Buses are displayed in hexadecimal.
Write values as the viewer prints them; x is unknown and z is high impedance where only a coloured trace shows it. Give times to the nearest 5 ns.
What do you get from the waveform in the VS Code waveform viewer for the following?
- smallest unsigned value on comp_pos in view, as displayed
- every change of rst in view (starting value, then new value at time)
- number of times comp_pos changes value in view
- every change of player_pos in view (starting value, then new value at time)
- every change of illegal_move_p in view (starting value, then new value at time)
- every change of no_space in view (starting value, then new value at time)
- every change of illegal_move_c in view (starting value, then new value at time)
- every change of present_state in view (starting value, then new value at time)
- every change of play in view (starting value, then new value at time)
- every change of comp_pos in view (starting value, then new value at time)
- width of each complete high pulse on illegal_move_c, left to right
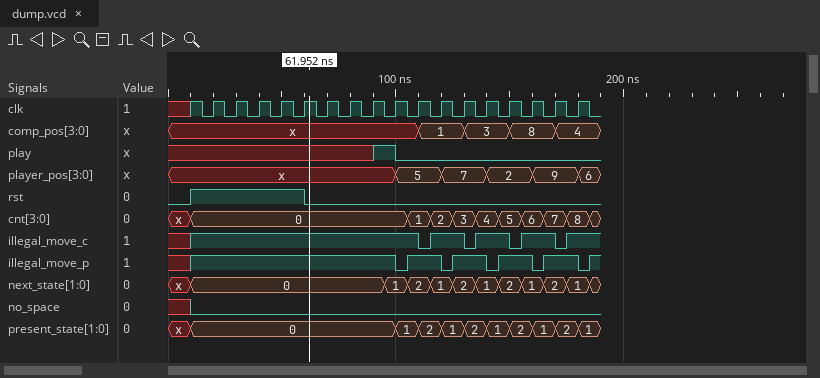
1
0, 1 at 10 ns, 0 at 60 ns
4
x, 5 at 100 ns, 7 at 120 ns, 2 at 140 ns, 9 at 160 ns, 6 at 180 ns
x, 1 at 10 ns, 0 at 100 ns, 1 at 105 ns, 0 at 120 ns, 1 at 125 ns, 0 at 140 ns, 1 at 145 ns, 0 at 160 ns, 1 at 165 ns, 0 at 180 ns, 1 at 185 ns
x, 0 at 10 ns
x, 1 at 10 ns, 0 at 110 ns, 1 at 115 ns, 0 at 130 ns, 1 at 135 ns, 0 at 150 ns, 1 at 155 ns, 0 at 170 ns, 1 at 175 ns
x, 0 at 10 ns, 1 at 100 ns, 2 at 110 ns, 1 at 120 ns, 2 at 130 ns, 1 at 140 ns, 2 at 150 ns, 1 at 160 ns, 2 at 170 ns, 1 at 180 ns
x, 1 at 90 ns, 0 at 100 ns
x, 1 at 110 ns, 3 at 130 ns, 8 at 150 ns, 4 at 170 ns
15 ns, 15 ns, 15 ns
